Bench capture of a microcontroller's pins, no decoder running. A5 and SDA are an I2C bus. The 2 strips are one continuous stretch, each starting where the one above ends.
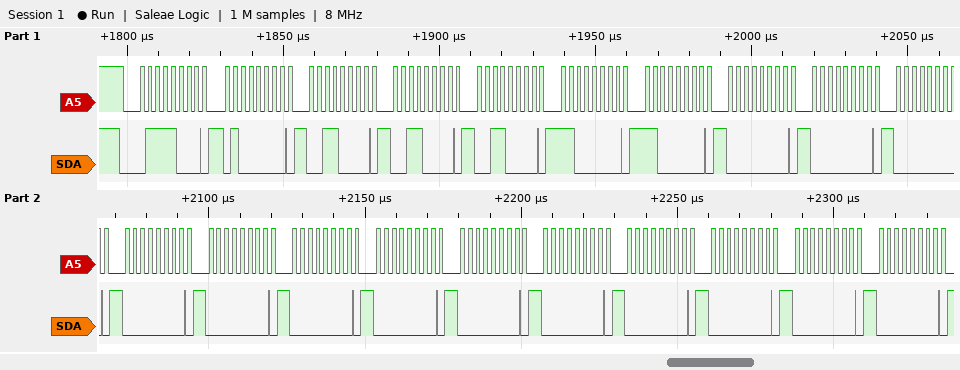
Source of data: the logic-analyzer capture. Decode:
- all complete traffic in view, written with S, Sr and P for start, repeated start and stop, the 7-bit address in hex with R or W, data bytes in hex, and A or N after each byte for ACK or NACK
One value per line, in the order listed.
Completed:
S 3CW A 40 A 30 A 30 A 30 A C0 A C0 A 00 A 00 A 00 A 00 A 00 A 00 A 00 A 00 A 00 A 00 A 00 A 00 A 00 A
